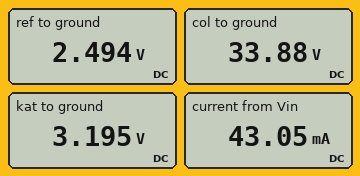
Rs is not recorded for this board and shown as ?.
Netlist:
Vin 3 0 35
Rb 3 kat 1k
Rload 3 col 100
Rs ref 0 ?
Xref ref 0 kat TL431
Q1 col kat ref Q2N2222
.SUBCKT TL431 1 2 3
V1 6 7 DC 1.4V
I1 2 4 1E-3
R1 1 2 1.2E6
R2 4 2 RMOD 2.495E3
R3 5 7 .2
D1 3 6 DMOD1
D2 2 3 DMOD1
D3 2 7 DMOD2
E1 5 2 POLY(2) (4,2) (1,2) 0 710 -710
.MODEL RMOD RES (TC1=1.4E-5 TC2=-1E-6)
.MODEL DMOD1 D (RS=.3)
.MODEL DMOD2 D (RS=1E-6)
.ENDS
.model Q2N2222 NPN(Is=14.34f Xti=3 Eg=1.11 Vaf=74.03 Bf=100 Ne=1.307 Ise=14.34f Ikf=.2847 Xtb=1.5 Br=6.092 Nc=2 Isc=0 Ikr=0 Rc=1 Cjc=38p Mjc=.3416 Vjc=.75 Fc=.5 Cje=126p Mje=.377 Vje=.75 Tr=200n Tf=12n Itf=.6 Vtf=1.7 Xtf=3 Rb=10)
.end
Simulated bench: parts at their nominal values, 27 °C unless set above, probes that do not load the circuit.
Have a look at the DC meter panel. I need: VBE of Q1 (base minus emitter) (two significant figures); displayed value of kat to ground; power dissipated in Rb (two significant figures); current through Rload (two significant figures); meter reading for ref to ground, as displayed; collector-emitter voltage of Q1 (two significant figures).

700 mV
3.195 V
1.0 W
11 mA
2.494 V
31 V
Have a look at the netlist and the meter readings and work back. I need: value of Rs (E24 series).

220 Ω
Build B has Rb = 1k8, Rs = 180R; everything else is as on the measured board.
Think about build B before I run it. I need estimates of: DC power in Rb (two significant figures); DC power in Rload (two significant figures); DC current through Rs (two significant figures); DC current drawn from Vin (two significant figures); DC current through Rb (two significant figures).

560 mW
19 mW
14 mA
31 mA
18 mA
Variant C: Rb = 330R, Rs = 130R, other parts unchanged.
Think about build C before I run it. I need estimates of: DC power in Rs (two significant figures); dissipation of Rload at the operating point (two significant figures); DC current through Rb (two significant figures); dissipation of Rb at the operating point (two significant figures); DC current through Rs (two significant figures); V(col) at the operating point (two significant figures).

48 mW
36 mW
96 mA
3.1 W
19 mA
33 V
